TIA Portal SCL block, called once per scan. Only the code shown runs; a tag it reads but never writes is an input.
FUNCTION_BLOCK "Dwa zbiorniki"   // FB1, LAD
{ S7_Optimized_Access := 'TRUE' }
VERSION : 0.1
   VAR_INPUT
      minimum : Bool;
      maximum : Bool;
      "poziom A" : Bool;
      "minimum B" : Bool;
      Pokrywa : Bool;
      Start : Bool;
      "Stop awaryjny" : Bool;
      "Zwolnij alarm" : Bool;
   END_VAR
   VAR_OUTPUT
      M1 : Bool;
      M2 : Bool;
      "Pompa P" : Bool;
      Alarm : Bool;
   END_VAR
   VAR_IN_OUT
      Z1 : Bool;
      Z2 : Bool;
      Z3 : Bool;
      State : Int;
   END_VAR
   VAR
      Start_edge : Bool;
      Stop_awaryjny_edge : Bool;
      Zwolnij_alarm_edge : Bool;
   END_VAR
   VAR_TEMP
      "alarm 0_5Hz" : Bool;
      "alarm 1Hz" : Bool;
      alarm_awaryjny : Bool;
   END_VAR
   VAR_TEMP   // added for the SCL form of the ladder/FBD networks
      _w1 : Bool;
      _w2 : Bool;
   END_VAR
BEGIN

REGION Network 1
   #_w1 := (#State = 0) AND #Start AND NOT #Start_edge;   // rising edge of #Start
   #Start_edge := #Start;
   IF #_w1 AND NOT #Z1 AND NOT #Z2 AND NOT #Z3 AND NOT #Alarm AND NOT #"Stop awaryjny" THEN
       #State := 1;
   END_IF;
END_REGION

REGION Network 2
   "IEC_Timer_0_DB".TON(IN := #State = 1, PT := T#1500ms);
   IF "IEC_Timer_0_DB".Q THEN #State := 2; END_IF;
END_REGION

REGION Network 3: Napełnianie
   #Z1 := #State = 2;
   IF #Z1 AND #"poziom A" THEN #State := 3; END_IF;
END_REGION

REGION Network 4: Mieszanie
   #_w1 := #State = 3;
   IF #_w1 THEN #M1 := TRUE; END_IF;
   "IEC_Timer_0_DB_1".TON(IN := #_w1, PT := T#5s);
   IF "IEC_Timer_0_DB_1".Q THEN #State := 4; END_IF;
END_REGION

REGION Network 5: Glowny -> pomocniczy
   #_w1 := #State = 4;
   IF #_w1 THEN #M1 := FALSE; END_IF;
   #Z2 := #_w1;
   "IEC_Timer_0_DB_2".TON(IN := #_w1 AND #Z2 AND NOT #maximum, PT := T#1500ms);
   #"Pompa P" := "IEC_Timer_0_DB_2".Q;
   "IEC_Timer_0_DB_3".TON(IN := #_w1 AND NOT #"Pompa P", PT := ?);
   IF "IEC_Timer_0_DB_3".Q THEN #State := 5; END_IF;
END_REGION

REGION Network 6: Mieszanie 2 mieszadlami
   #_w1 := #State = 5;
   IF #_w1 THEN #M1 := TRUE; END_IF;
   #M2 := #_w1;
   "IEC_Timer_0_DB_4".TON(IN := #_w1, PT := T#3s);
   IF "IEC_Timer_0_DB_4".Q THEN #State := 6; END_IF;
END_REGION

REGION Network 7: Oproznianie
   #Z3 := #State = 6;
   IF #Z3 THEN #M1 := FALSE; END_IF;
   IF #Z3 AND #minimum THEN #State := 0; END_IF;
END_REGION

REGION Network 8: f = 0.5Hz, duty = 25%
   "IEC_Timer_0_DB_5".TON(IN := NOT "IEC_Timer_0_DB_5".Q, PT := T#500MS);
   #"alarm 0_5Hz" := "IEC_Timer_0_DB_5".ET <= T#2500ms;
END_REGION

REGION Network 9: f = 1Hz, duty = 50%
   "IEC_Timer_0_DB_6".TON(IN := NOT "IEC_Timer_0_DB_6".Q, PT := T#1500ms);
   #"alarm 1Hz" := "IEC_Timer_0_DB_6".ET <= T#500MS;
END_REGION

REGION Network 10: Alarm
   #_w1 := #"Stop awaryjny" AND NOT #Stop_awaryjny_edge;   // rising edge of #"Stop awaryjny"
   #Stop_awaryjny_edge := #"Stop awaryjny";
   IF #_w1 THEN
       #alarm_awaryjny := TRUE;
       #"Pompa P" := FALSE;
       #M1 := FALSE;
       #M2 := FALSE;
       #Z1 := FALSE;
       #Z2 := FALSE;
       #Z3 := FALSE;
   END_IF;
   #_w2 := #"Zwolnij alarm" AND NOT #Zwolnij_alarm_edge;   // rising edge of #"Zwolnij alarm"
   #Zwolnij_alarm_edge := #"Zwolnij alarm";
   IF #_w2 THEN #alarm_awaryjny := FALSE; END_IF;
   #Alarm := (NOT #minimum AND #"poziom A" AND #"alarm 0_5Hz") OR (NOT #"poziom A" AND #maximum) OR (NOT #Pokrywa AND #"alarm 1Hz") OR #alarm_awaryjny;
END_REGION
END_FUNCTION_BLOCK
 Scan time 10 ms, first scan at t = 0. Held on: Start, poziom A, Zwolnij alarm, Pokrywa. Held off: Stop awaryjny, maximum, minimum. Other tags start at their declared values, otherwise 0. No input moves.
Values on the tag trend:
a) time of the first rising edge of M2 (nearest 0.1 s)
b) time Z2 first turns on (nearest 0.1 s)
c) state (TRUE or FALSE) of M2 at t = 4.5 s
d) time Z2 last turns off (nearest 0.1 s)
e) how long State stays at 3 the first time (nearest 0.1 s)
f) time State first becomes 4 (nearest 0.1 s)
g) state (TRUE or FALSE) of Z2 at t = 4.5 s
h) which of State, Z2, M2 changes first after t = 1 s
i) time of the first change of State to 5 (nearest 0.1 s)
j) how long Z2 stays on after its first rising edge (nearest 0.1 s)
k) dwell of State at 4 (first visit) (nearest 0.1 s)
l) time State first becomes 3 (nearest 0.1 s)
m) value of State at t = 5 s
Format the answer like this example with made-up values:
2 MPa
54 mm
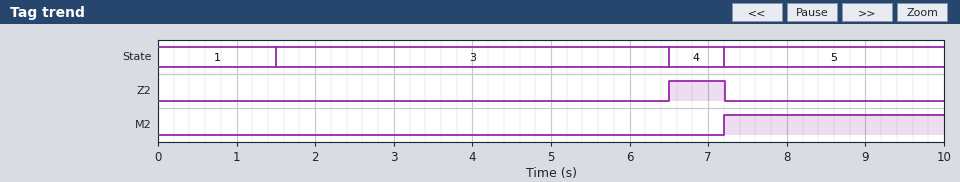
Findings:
7.2 s
6.5 s
FALSE
7.2 s
5.0 s
6.5 s
FALSE
State
7.2 s
0.7 s
0.7 s
1.5 s
3
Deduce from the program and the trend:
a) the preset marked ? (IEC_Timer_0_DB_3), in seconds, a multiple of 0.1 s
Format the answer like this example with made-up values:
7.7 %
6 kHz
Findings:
0.7 s
